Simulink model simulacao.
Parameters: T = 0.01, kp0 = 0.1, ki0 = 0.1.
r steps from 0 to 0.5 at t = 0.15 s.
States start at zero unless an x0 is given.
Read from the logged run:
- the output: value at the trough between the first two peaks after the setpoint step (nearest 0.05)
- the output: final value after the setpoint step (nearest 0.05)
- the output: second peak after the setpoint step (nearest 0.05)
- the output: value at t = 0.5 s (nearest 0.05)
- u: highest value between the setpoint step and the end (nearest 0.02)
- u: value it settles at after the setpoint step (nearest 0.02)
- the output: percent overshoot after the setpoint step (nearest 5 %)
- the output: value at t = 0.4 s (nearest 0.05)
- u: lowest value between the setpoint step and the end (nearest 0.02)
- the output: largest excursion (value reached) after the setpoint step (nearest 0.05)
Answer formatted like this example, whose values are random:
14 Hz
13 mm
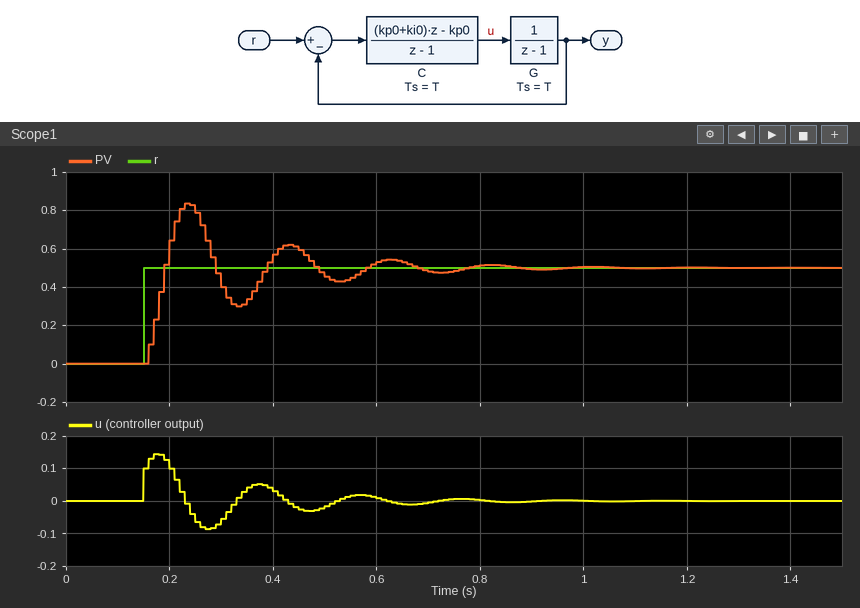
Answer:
0.30
0.50
0.60
0.45
0.14
0.00
65 %
0.55
-0.08
0.85
